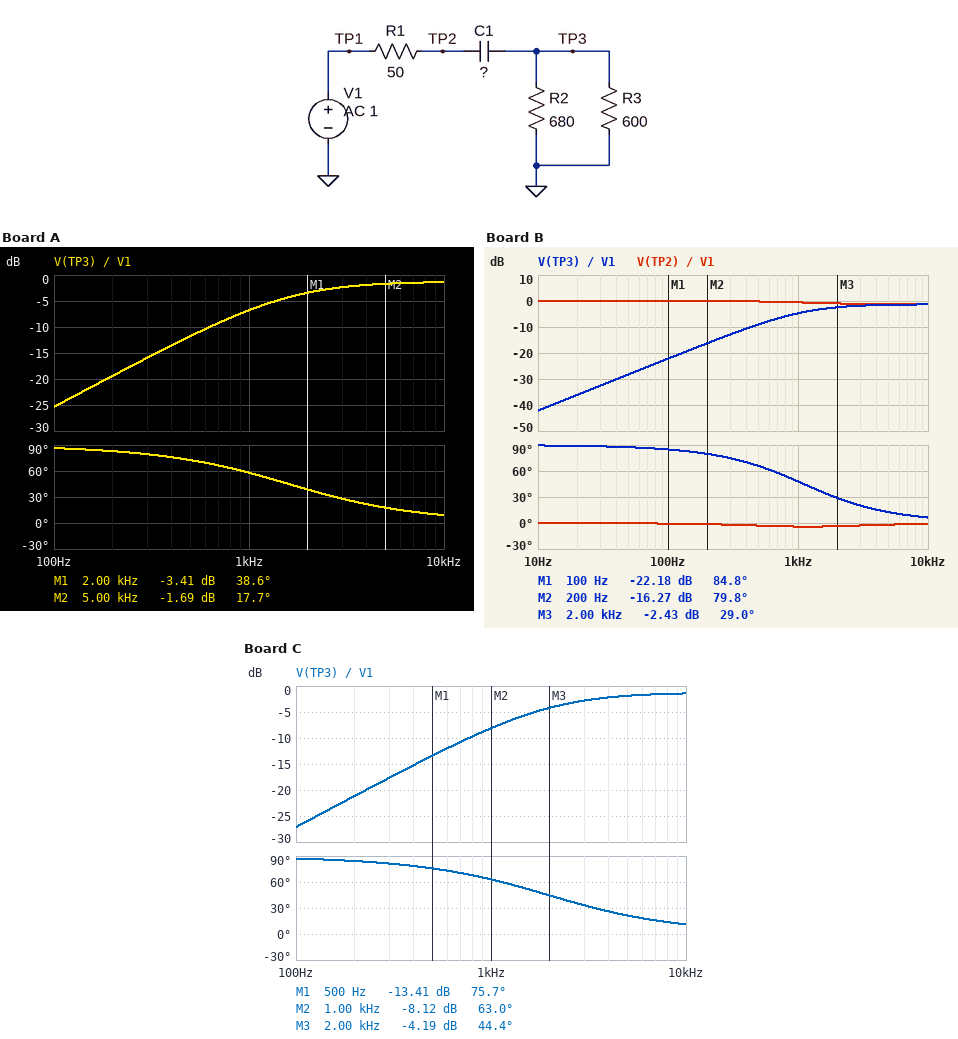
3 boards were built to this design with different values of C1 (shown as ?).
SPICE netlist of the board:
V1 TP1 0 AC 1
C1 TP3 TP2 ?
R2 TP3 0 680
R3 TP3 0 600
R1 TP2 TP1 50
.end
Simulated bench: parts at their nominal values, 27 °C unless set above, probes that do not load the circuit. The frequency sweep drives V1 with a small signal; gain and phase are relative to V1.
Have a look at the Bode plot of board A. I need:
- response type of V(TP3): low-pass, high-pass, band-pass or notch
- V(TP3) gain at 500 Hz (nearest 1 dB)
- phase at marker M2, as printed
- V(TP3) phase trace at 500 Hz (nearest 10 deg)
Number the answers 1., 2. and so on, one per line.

1. high-pass
2. -12 dB
3. 17.7 deg
4. 70 deg
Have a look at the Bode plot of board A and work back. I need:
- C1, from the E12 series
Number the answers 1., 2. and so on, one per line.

1. 270 nF
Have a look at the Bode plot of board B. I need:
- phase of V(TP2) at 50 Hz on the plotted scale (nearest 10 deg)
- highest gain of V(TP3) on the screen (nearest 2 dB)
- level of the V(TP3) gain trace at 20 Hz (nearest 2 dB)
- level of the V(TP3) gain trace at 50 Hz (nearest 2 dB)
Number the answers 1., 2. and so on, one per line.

1. 0 deg
2. -2 dB
3. -36 dB
4. -28 dB
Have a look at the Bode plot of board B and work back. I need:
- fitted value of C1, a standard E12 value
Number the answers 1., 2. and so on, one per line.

1. 390 nF
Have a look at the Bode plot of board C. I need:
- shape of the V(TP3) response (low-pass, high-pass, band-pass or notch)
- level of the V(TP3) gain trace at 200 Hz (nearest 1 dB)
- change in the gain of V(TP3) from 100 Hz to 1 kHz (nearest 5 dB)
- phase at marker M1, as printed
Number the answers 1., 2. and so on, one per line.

1. high-pass
2. -21 dB
3. 20 dB
4. 75.7 deg
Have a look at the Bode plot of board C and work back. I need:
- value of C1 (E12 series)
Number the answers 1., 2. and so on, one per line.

1. 220 nF
